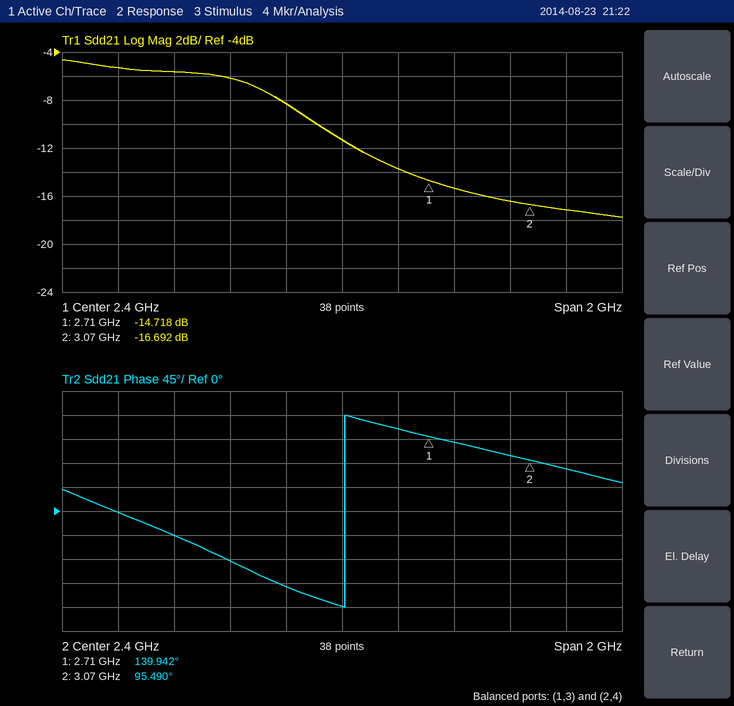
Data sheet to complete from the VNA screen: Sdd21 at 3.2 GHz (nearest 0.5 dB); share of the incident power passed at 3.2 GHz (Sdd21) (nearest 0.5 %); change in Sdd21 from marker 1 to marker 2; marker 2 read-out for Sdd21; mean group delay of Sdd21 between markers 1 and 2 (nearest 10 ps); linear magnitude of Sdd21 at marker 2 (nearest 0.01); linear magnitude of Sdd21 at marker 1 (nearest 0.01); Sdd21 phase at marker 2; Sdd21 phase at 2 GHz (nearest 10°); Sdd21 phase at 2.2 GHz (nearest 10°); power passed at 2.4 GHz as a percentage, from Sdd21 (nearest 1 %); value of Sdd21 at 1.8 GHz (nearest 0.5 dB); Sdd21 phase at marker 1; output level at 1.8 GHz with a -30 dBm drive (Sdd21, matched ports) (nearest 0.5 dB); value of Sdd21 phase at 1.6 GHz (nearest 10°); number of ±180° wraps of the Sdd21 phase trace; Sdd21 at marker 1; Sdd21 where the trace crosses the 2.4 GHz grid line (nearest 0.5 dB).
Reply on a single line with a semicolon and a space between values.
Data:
-17.0 dB; 2.0 %; -1.974 dB; -16.692 dB; 340 ps; 0.15; 0.18; 95.490°; -90°; -140°; 7 %; -5.5 dB; 139.942°; -35.5 dBm; 0°; 1; -14.718 dB; -11.5 dB
